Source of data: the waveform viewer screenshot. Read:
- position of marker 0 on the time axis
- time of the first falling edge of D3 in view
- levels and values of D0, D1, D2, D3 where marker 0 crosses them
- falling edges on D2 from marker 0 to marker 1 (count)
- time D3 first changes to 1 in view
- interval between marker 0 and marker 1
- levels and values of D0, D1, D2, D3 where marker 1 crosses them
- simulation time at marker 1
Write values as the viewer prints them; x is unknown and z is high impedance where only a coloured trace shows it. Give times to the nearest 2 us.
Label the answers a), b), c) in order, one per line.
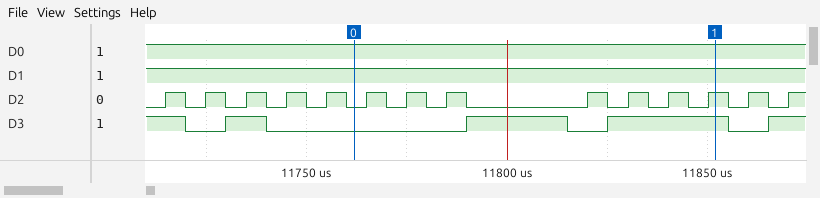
a) 11762 us
b) 11720 us
c) D0=1, D1=1, D2=0, D3=0
d) 6
e) 11730 us
f) 90 us
g) D0=1, D1=1, D2=1, D3=1
h) 11852 us
